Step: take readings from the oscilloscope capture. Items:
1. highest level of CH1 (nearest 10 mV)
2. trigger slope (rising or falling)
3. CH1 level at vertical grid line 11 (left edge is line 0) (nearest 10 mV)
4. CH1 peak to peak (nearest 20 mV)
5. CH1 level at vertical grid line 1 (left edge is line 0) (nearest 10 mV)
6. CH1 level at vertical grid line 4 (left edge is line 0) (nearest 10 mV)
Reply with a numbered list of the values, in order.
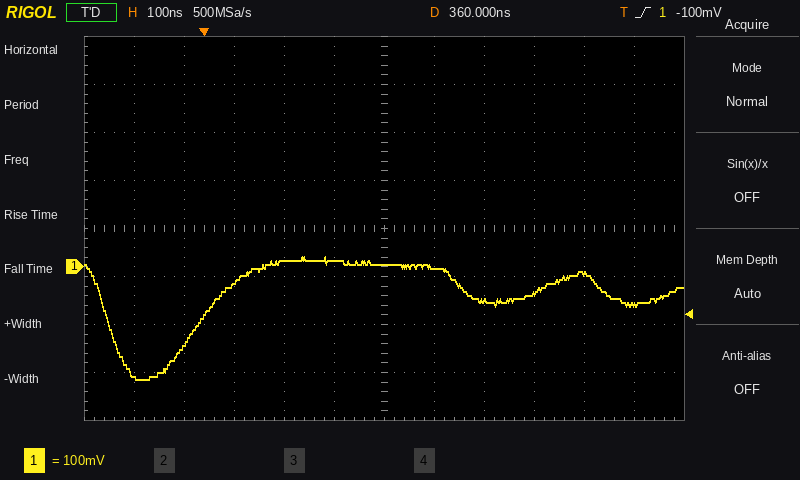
1. 20 mV
2. rising
3. -80 mV
4. 260 mV
5. -230 mV
6. 10 mV
